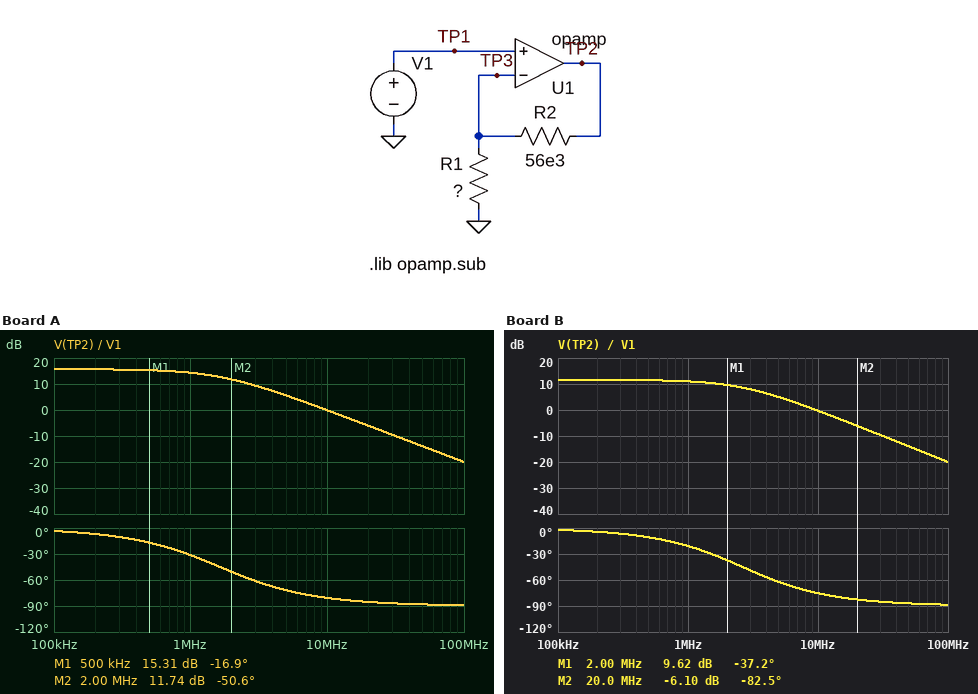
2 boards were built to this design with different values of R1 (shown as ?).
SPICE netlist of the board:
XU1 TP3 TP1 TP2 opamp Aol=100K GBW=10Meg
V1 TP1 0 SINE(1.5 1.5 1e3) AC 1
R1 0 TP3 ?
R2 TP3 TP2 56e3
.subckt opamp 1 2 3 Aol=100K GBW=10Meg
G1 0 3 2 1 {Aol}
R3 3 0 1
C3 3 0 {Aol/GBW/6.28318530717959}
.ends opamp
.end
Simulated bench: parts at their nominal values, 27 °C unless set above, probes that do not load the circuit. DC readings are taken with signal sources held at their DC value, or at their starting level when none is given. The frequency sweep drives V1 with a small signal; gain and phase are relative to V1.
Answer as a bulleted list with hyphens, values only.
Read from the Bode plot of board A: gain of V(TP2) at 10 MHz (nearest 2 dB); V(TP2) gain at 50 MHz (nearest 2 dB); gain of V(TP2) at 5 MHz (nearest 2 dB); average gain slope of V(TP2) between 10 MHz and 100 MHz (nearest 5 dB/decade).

- 0 dB
- -14 dB
- 6 dB
- -20 dB/decade
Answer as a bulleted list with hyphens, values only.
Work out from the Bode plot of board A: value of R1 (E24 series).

- 11 kΩ
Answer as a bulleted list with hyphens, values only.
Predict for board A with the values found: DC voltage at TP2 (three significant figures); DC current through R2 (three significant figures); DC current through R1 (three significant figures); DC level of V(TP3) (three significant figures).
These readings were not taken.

- 9.14 V
- 136 µA
- 136 µA
- 1.50 V
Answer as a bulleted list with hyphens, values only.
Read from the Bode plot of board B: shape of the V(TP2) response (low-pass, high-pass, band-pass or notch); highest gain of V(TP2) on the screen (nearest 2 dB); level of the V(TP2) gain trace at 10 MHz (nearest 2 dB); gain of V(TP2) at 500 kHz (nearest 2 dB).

- low-pass
- 12 dB
- 0 dB
- 12 dB
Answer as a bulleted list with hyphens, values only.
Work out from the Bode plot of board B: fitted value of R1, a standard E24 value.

- 20 kΩ
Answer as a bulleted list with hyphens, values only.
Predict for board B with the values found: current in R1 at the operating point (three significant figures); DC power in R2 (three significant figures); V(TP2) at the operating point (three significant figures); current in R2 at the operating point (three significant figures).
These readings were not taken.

- 75.0 µA
- 315 µW
- 5.70 V
- 75.0 µA
